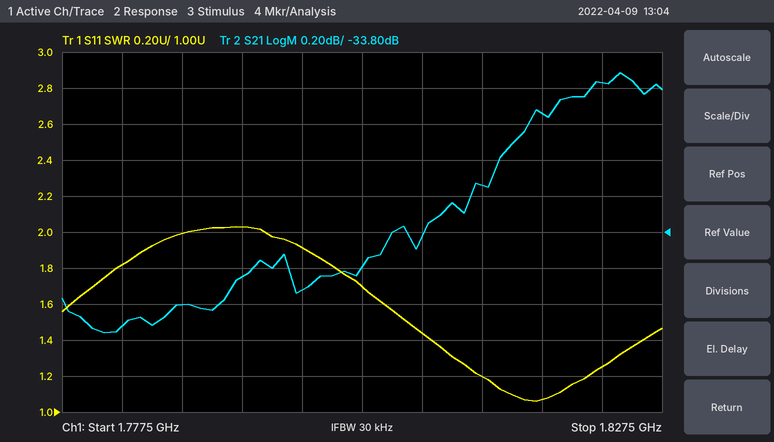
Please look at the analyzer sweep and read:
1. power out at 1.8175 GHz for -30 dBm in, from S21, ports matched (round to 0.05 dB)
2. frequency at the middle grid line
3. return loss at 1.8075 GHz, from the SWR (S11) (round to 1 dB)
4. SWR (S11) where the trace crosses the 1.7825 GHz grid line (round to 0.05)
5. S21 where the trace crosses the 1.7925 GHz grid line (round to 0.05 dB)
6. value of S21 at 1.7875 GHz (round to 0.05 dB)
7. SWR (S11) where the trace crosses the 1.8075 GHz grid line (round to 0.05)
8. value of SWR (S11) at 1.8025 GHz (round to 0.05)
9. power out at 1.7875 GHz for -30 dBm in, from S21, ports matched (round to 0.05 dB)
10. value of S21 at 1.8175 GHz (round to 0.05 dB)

-63.15 dBm
1.8025 GHz
15 dB
1.80
-34.05 dB
-34.20 dB
1.45
1.70
-64.20 dBm
-33.15 dB
